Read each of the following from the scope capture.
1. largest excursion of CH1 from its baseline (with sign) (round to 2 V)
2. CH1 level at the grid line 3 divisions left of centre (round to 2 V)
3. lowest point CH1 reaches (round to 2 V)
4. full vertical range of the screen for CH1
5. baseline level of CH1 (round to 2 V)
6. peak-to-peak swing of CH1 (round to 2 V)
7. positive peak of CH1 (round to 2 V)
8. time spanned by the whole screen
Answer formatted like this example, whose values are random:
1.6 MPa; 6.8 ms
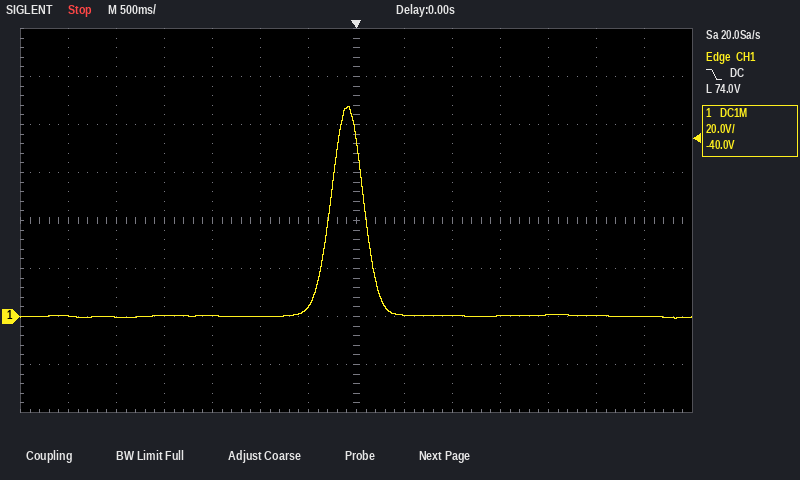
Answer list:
+88 V; 0 V; 0 V; 160 V; 0 V; 88 V; 88 V; 7 s
